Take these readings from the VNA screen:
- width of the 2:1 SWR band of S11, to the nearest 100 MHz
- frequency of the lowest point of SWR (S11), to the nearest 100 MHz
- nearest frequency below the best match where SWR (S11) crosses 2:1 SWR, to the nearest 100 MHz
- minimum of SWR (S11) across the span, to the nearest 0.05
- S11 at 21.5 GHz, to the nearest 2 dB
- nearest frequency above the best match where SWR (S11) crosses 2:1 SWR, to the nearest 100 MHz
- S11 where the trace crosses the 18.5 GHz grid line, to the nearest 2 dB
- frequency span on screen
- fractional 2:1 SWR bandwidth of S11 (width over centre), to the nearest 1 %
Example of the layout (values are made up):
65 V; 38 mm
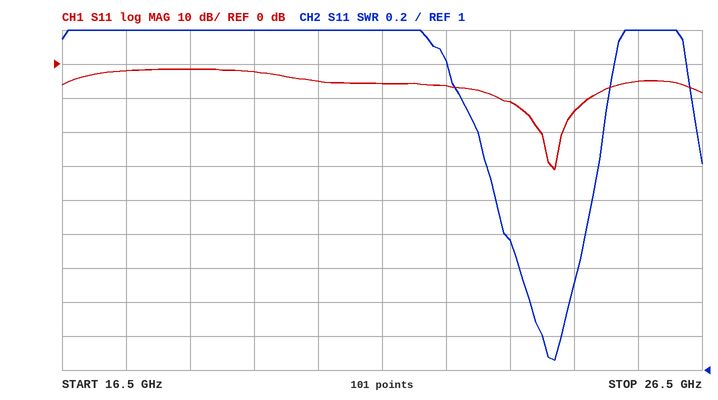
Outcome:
1.5 GHz; 24.2 GHz; 23.3 GHz; 1.05; -6 dB; 24.8 GHz; -2 dB; 10 GHz; 6 %
